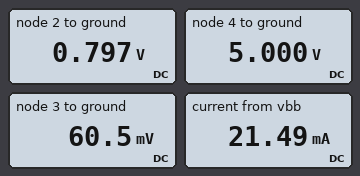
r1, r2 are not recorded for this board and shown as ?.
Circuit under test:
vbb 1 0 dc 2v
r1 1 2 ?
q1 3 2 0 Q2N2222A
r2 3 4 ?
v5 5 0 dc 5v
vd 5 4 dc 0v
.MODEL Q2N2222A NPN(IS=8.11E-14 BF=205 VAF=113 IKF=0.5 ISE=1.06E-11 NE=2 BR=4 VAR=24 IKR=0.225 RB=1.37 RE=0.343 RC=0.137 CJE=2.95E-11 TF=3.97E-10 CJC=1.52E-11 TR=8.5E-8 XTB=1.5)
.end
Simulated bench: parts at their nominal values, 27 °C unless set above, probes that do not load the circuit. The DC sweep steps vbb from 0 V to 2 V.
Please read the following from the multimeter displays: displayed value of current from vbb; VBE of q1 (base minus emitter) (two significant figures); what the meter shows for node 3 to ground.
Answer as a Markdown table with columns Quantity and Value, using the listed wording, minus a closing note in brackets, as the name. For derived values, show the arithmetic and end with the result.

| Quantity | Value |
|---|---|
| displayed value of current from vbb | 21.49 mA |
| VBE of q1 (base minus emitter) | 797 mV = 800 mV |
| what the meter shows for node 3 to ground | 60.5 mV |
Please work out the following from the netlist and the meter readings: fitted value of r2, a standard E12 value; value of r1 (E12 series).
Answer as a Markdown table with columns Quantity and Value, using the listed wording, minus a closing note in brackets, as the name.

| Quantity | Value |
|---|---|
| fitted value of r2, a standard E12 value | 82 Ω |
| value of r1 | 56 Ω |
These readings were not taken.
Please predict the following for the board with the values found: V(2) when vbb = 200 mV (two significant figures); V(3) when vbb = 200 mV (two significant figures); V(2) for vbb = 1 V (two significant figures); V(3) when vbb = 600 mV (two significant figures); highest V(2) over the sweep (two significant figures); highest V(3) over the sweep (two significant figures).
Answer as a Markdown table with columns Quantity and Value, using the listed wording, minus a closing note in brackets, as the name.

| Quantity | Value |
|---|---|
| V(2) when vbb = 200 mV | 200 mV |
| V(3) when vbb = 200 mV | 5.0 V |
| V(2) for vbb = 1 V | 750 mV |
| V(3) when vbb = 600 mV | 4.9 V |
| highest V(2) over the sweep | 800 mV |
| highest V(3) over the sweep | 5.0 V |
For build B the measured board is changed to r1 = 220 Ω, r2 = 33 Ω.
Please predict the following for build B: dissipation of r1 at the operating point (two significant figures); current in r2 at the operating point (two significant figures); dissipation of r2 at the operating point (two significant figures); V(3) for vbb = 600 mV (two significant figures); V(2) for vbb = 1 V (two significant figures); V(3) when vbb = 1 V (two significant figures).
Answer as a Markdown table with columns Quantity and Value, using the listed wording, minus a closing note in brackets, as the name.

| Quantity | Value |
|---|---|
| dissipation of r1 at the operating point | 6.5 mW |
| current in r2 at the operating point | 150 mA |
| dissipation of r2 at the operating point | 720 mW |
| V(3) for vbb = 600 mV | 5.0 V |
| V(2) for vbb = 1 V | 790 mV |
| V(3) when vbb = 1 V | 280 mV |
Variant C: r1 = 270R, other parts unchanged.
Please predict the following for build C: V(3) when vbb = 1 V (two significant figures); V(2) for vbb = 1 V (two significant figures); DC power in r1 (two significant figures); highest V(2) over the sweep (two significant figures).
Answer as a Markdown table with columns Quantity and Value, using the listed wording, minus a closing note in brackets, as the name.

| Quantity | Value |
|---|---|
| V(3) when vbb = 1 V | 120 mV |
| V(2) for vbb = 1 V | 730 mV |
| DC power in r1 | 5.8 mW |
| highest V(2) over the sweep | 750 mV |
